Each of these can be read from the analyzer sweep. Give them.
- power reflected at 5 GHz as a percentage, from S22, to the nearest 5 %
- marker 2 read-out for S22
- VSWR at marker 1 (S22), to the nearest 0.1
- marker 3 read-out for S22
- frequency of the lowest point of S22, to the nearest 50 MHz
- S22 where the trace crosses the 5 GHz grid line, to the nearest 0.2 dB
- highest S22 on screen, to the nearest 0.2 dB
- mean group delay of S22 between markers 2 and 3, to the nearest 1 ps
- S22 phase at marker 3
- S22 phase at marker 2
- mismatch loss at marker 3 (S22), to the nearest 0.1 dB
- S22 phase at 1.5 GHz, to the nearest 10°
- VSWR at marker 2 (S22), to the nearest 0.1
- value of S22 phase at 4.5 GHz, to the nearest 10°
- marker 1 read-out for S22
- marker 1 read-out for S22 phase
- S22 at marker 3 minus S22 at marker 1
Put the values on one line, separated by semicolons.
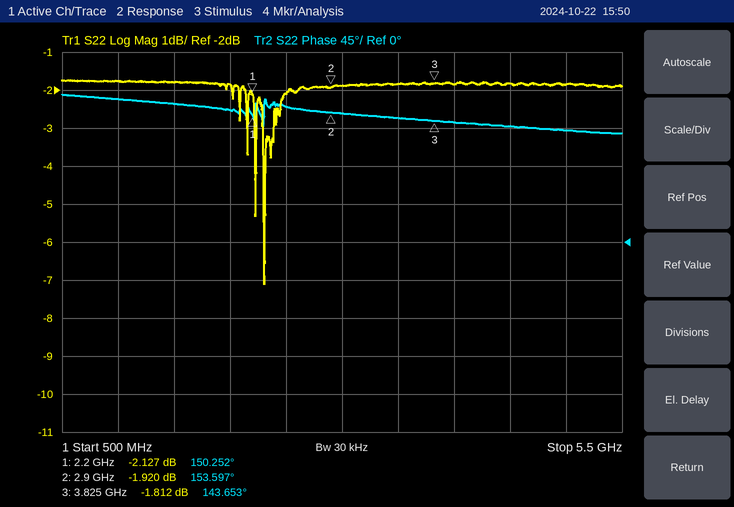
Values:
65 %; -1.920 dB; 8.2; -1.812 dB; 2.30 GHz; -1.8 dB; -1.8 dB; 30 ps; 143.653°; 153.597°; 4.7 dB; 160°; 9.1; 140°; -2.127 dB; 150.252°; 0.315 dB
